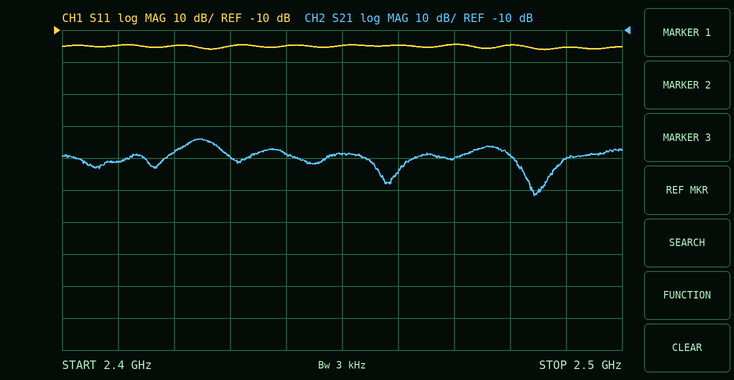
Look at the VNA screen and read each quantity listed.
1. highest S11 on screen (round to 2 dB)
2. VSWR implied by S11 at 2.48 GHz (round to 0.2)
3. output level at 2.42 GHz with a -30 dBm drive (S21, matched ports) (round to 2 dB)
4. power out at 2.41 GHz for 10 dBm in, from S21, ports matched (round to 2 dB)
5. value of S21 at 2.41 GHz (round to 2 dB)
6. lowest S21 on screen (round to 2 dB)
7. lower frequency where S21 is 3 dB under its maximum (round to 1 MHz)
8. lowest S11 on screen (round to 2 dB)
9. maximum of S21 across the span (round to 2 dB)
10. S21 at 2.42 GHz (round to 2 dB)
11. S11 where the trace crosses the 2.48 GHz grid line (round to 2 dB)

-14 dB
1.4
-78 dBm
-42 dBm
-52 dB
-62 dB
2.421 GHz
-16 dB
-44 dB
-48 dB
-14 dB
